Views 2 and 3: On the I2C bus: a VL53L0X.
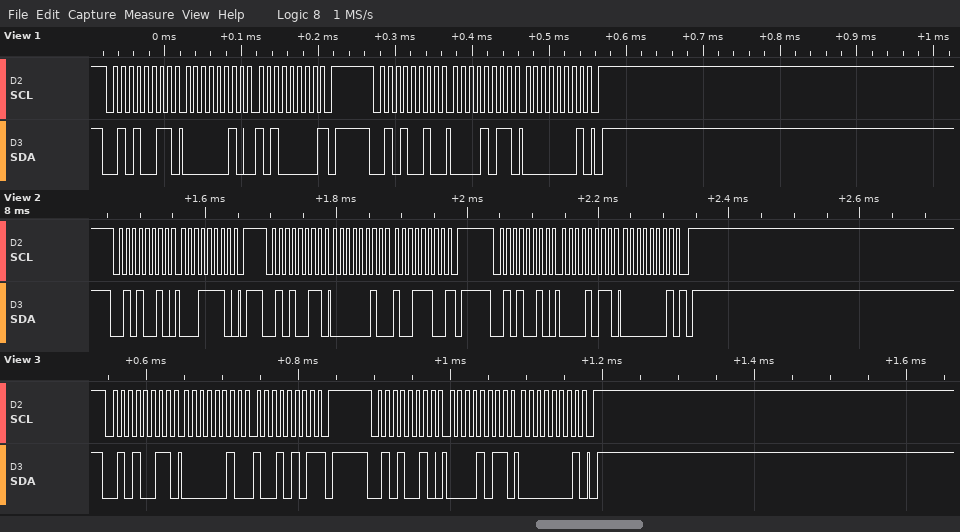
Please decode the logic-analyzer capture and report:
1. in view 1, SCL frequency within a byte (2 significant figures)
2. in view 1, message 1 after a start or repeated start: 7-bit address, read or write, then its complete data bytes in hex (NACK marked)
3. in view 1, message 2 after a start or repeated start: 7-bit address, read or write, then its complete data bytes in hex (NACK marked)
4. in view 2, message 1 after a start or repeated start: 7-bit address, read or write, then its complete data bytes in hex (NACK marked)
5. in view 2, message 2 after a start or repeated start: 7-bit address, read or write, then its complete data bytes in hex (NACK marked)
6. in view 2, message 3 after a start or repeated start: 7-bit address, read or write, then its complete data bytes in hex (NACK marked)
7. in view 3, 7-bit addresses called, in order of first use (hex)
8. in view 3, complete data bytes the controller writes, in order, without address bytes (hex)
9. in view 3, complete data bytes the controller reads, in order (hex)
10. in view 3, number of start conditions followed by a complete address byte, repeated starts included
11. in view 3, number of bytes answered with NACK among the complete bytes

100 kHz
0x29 read: 02 A0 NACK
0x29 write: 0B 01
0x29 write: 1E
0x29 read: 02 9C NACK
0x29 write: 0B 01
0x29
0B 01
02 95
2
1
